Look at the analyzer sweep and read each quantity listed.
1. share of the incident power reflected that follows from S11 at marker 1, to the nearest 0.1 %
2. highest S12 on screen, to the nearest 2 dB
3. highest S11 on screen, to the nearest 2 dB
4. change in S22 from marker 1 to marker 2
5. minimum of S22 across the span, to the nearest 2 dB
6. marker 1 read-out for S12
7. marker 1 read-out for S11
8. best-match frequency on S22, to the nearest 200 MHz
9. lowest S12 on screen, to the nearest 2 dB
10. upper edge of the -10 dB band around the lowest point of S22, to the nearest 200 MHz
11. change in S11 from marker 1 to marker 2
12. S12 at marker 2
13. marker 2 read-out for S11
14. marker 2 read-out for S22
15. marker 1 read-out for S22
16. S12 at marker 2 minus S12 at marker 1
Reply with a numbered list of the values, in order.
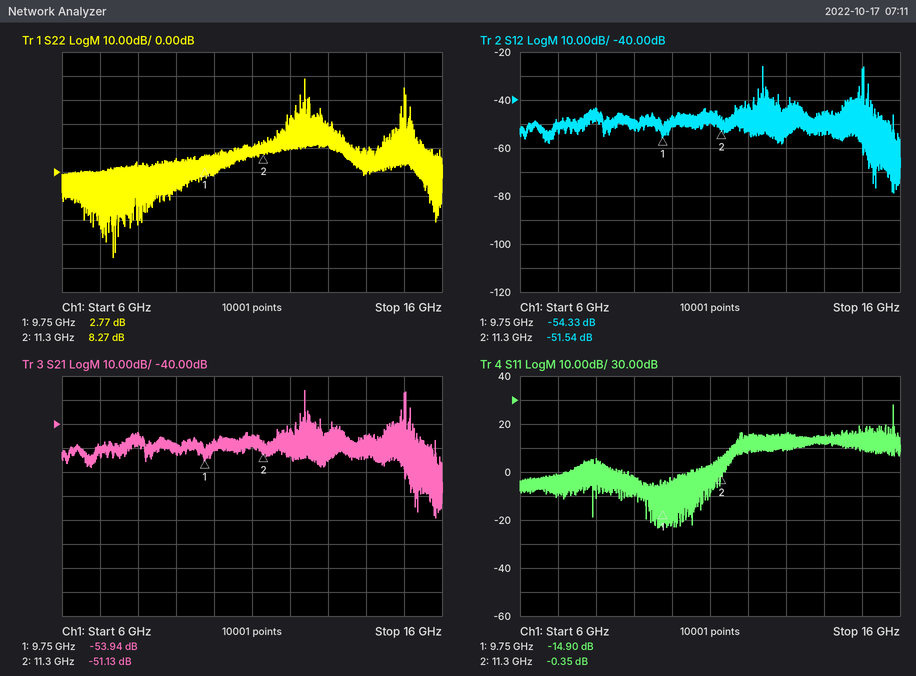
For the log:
1. 3.2 %
2. -26 dB
3. 28 dB
4. 5.50 dB
5. -36 dB
6. -54.33 dB
7. -14.90 dB
8. 7.4 GHz
9. -78 dB
10. 7.4 GHz
11. 14.55 dB
12. -51.54 dB
13. -0.35 dB
14. 8.27 dB
15. 2.77 dB
16. 2.79 dB
